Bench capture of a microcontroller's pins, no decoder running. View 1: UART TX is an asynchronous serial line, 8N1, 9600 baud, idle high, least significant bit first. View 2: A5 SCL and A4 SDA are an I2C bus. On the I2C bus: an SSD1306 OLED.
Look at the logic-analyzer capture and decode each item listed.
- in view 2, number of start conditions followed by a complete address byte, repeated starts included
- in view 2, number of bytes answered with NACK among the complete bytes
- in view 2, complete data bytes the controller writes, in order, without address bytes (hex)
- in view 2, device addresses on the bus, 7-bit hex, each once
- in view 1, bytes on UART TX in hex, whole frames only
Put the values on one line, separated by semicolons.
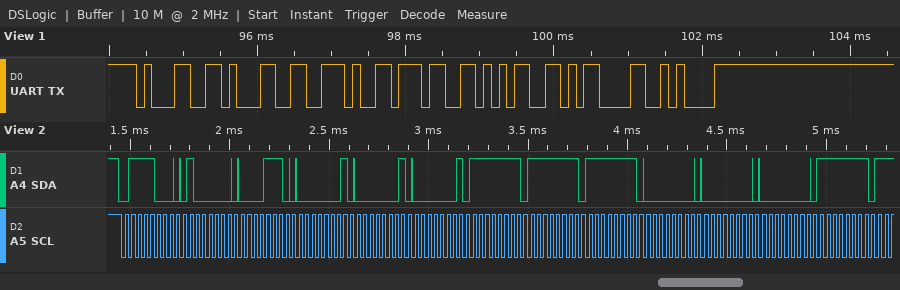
1; 0; 40 0E 01 01 01 FF FF FF 00 00 00 FF; 0x3C; 31 31 2E 37 35 0D 0A
